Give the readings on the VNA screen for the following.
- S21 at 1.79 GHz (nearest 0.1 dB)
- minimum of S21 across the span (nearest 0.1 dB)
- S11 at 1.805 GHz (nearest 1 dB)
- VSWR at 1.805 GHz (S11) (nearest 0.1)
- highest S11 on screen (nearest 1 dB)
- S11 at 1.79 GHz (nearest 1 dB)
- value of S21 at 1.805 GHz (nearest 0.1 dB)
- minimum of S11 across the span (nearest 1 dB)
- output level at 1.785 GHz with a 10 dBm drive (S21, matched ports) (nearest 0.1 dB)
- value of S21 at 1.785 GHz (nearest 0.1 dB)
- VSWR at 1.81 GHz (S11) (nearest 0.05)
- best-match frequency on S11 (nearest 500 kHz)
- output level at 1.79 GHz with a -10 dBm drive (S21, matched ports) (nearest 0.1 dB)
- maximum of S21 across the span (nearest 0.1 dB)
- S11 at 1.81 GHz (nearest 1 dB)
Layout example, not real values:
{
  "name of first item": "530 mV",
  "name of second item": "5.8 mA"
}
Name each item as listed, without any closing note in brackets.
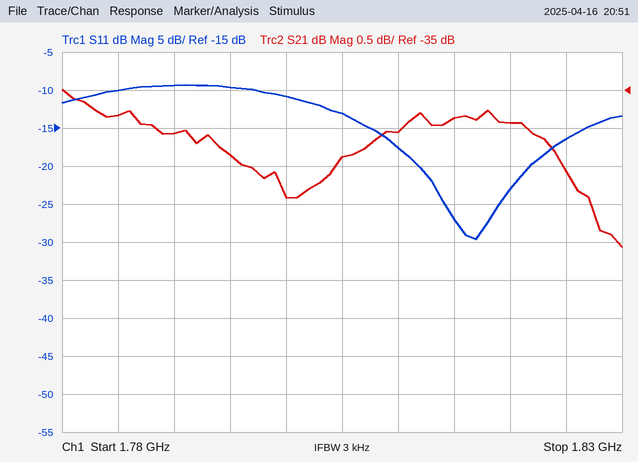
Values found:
{
  "S21 at 1.79 GHz": "-35.6 dB",
  "minimum of S21 across the span": "-37.1 dB",
  "S11 at 1.805 GHz": "-13 dB",
  "VSWR at 1.805 GHz (S11)": "1.6",
  "highest S11 on screen": "-9 dB",
  "S11 at 1.79 GHz": "-9 dB",
  "value of S21 at 1.805 GHz": "-35.9 dB",
  "minimum of S11 across the span": "-30 dB",
  "output level at 1.785 GHz with a 10 dBm drive (S21, matched ports)": "-25.3 dBm",
  "value of S21 at 1.785 GHz": "-35.3 dB",
  "VSWR at 1.81 GHz (S11)": "1.30",
  "best-match frequency on S11": "1.8170 GHz",
  "output level at 1.79 GHz with a -10 dBm drive (S21, matched ports)": "-45.6 dBm",
  "maximum of S21 across the span": "-35.0 dB",
  "S11 at 1.81 GHz": "-18 dB"
}
